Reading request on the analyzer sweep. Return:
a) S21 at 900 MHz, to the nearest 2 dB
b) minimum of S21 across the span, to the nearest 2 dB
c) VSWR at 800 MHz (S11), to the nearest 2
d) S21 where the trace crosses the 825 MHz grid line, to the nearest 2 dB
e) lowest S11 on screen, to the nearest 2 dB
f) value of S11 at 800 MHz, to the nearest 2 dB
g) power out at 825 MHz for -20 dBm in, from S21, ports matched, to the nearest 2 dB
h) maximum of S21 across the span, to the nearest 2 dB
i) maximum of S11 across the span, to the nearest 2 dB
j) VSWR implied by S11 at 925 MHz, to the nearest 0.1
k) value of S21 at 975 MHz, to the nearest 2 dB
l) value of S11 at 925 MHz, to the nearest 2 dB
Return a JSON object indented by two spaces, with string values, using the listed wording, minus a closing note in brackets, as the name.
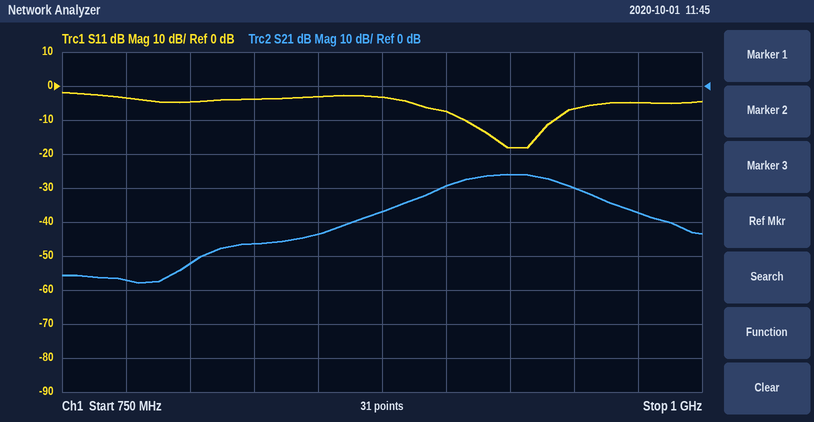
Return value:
{
  "S21 at 900 MHz, to the nearest 2 dB": "-30 dB",
  "minimum of S21 across the span, to the nearest 2 dB": "-58 dB",
  "VSWR at 800 MHz (S11), to the nearest 2": "4",
  "S21 where the trace crosses the 825 MHz grid line, to the nearest 2 dB": "-46 dB",
  "lowest S11 on screen, to the nearest 2 dB": "-18 dB",
  "value of S11 at 800 MHz, to the nearest 2 dB": "-4 dB",
  "power out at 825 MHz for -20 dBm in, from S21, ports matched, to the nearest 2 dB": "-66 dBm",
  "maximum of S21 across the span, to the nearest 2 dB": "-26 dB",
  "maximum of S11 across the span, to the nearest 2 dB": "-2 dB",
  "VSWR implied by S11 at 925 MHz, to the nearest 0.1": "1.3",
  "value of S21 at 975 MHz, to the nearest 2 dB": "-38 dB",
  "value of S11 at 925 MHz, to the nearest 2 dB": "-18 dB"
}
